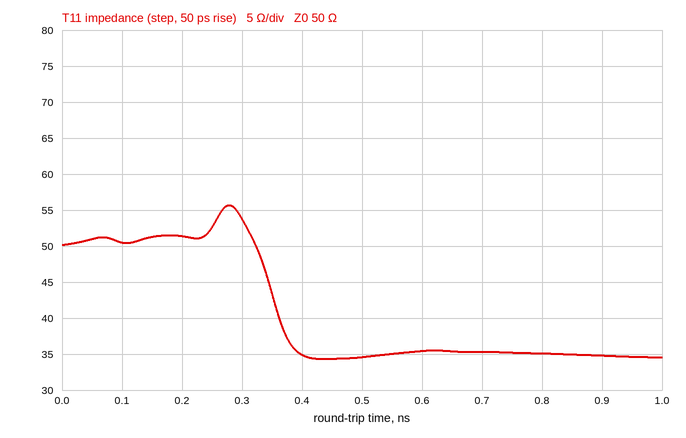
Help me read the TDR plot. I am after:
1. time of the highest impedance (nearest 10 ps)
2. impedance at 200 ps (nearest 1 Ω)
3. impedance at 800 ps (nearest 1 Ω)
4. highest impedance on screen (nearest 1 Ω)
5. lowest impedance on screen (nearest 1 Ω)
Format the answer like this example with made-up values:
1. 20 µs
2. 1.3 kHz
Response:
1. 280 ps
2. 51 Ω
3. 35 Ω
4. 56 Ω
5. 34 Ω
